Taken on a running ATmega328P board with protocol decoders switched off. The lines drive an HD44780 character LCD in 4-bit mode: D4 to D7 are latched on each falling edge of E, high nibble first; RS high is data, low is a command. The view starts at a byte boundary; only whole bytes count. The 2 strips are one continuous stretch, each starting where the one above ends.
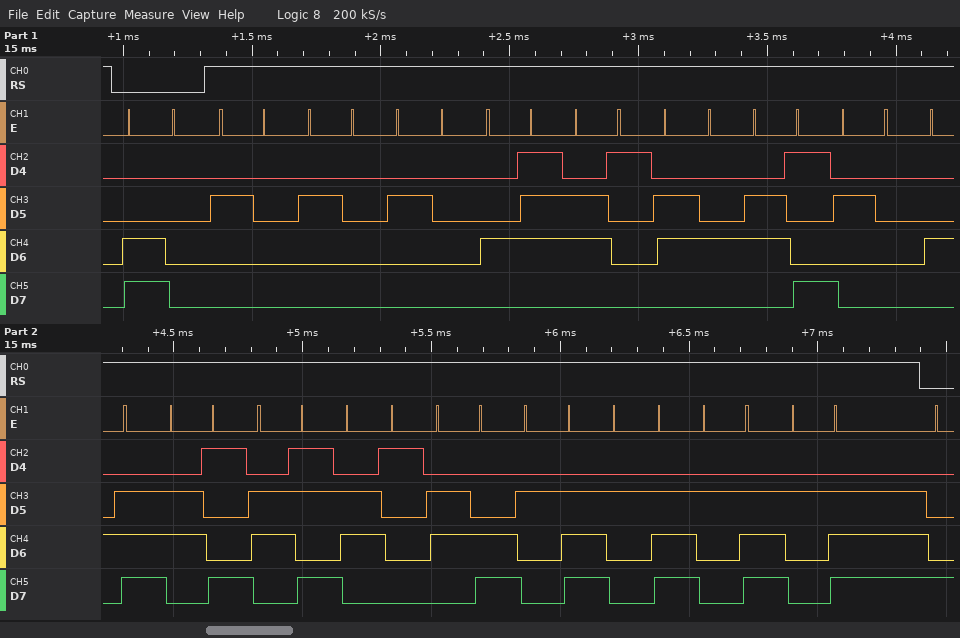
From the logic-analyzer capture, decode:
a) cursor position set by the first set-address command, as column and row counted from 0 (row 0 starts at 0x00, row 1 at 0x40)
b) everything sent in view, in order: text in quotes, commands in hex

column 0, row 1
0xC0 "   Gadi Nikal...."
